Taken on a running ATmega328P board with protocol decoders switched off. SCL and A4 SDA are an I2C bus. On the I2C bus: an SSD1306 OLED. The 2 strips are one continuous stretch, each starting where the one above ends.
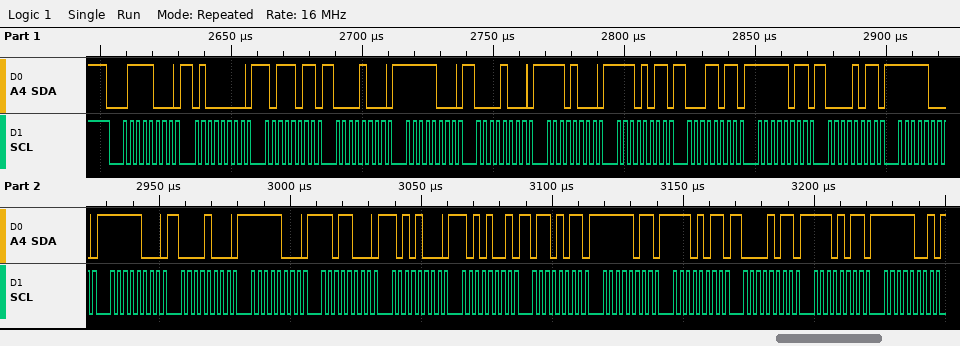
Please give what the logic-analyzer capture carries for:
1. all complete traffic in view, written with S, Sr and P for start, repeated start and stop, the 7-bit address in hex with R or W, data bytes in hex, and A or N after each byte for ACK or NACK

S 3CW A 40 A BB A 08 A F8 A 08 A E8 A EB A 1B A FB A 0B A F8 A F8 A 08 A F8 A D8 A A8 A A9 A 6B A FB A EB A 0B A EB A F9 A
